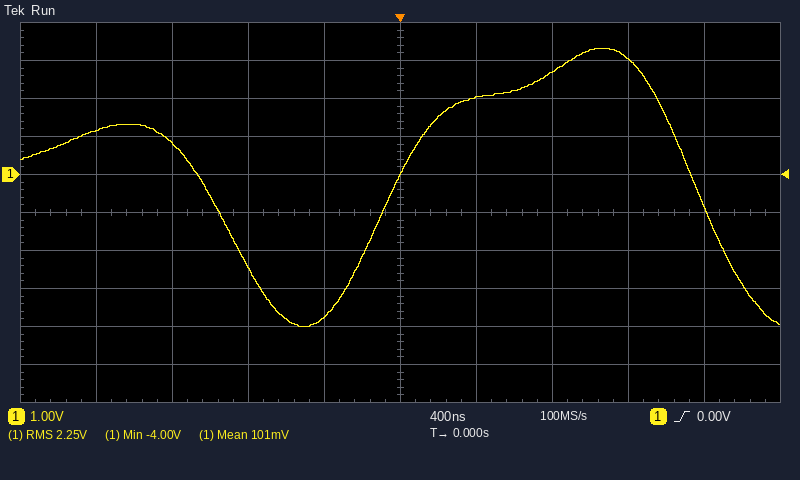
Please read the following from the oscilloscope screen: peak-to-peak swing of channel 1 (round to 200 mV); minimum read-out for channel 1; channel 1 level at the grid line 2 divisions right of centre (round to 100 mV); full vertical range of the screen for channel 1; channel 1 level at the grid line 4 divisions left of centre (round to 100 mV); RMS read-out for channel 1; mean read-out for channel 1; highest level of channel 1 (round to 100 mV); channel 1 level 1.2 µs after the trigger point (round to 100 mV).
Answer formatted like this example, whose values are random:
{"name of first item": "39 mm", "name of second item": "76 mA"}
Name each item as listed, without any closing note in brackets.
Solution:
{"peak-to-peak swing of channel 1": "7.4 V", "minimum read-out for channel 1": "-4.00 V", "channel 1 level at the grid line 2 divisions right of centre": "2.7 V", "full vertical range of the screen for channel 1": "10 V", "channel 1 level at the grid line 4 divisions left of centre": "1.2 V", "RMS read-out for channel 1": "2.25 V", "mean read-out for channel 1": "101 mV", "highest level of channel 1": "3.3 V", "channel 1 level 1.2 µs after the trigger point": "3.0 V"}
